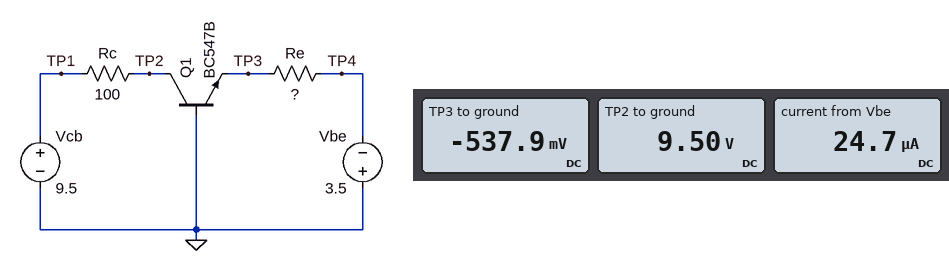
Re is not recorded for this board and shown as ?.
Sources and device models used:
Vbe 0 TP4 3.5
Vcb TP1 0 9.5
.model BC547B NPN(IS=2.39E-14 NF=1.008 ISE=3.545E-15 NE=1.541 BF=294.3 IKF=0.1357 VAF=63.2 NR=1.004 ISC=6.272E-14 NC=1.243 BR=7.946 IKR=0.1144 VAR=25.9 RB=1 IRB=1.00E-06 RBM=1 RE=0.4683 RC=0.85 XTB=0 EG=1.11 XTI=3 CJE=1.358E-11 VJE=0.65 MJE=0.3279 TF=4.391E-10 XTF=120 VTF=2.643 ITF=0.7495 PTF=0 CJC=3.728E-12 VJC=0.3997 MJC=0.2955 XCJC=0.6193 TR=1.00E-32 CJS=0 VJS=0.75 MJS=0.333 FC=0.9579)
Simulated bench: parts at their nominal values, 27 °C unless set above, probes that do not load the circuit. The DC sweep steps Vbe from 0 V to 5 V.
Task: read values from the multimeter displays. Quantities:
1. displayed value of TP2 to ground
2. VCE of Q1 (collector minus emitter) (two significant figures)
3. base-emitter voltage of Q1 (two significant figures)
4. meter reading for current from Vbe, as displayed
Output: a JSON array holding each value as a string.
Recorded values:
["9.50 V", "10 V", "540 mV", "24.7 µA"]
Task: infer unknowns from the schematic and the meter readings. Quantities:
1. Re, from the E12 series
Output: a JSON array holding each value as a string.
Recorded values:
["120 kΩ"]
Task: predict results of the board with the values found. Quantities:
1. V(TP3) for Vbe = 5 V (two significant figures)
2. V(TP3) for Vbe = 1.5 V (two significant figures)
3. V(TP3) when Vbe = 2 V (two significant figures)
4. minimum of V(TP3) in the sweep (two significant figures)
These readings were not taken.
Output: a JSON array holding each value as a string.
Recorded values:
["-550 mV", "-510 mV", "-520 mV", "-550 mV"]
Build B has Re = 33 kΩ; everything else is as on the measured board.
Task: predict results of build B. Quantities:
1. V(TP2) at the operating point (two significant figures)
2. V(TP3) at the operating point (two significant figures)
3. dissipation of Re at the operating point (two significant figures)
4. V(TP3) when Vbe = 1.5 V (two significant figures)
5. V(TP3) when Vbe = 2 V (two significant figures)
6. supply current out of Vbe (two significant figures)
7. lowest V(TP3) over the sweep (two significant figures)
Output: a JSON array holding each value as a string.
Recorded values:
["9.5 V", "-570 mV", "260 µW", "-540 mV", "-550 mV", "89 µA", "-580 mV"]
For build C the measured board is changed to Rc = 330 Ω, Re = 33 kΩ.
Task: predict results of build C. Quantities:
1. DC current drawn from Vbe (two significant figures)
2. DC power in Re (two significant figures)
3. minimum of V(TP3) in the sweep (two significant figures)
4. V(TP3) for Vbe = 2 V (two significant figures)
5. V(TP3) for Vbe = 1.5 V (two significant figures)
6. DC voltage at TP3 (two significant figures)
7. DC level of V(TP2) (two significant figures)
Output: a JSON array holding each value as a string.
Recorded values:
["89 µA", "260 µW", "-580 mV", "-550 mV", "-540 mV", "-570 mV", "9.5 V"]
